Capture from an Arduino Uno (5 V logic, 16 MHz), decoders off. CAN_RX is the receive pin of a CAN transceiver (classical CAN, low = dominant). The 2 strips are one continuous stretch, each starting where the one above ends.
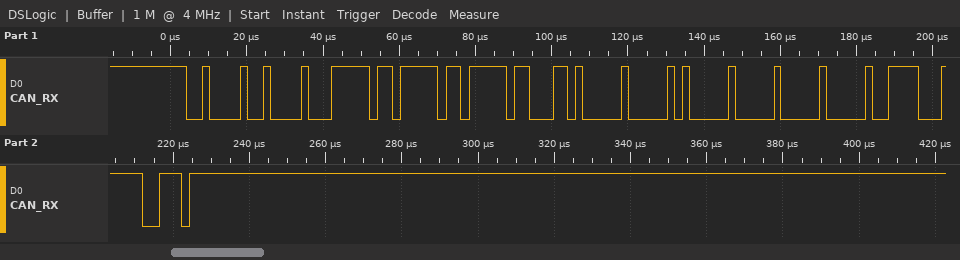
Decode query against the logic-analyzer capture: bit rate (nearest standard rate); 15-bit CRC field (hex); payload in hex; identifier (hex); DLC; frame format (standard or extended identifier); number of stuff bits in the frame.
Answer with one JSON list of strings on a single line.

["500 kbit/s", "0x78FB", "FE FE FE 34 00 40 00 00", "0x212", "8", "standard", "10"]
